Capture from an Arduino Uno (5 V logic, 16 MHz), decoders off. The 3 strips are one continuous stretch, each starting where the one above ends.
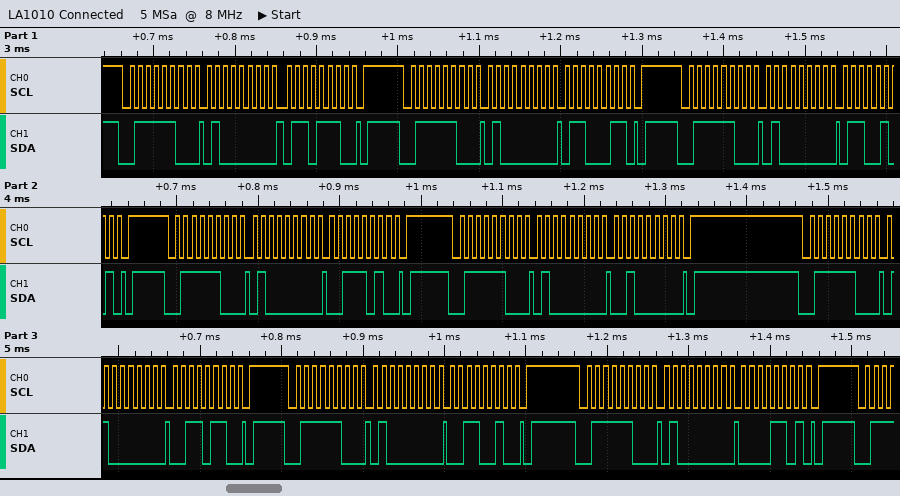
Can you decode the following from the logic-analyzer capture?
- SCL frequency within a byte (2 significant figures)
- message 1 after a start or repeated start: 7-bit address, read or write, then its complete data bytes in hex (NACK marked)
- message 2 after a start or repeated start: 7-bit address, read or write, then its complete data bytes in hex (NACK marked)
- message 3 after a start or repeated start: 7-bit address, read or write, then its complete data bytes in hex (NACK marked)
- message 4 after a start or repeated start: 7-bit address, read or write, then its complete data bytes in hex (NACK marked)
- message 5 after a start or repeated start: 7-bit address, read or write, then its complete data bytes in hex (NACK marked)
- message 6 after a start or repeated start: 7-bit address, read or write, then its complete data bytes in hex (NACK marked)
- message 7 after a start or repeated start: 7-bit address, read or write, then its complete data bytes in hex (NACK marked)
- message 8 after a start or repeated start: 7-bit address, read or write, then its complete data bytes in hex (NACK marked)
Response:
100 kHz
0x3E write: 40 6E
0x3E write: 40 63
0x3E write: 40 65
0x3E write: 40 3A
0x3E write: 40 20
0x3E write: 40 36
0x3E write: 40 32
0x3E write: 40 0D
